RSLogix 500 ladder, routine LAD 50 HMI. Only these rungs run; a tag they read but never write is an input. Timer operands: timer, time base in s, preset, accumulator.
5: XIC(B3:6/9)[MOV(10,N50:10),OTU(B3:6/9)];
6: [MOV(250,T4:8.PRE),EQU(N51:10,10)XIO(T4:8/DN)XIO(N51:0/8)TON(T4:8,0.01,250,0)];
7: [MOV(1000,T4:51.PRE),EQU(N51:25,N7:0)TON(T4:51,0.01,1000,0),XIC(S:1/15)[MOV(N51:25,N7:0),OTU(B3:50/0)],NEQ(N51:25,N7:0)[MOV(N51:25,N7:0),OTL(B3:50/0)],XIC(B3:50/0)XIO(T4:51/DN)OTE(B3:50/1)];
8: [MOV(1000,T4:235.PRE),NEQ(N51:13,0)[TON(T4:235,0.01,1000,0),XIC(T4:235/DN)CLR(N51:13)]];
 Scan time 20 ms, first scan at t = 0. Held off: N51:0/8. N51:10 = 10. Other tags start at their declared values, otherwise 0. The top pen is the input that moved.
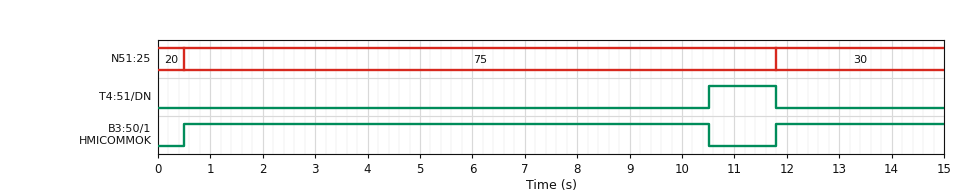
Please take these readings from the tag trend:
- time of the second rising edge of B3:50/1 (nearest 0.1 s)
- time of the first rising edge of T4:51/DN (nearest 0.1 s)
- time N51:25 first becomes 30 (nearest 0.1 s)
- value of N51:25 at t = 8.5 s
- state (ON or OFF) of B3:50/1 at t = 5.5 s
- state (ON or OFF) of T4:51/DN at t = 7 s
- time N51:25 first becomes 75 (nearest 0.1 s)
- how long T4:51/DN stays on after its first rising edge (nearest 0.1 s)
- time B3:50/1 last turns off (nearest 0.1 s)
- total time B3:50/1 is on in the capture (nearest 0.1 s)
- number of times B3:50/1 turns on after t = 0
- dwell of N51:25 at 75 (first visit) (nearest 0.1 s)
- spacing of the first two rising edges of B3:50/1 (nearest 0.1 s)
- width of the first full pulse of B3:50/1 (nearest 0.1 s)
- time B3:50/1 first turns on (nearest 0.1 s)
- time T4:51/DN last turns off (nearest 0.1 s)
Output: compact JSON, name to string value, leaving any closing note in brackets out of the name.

{"time of the second rising edge of B3:50/1": "11.8 s", "time of the first rising edge of T4:51/DN": "10.5 s", "time N51:25 first becomes 30": "11.8 s", "value of N51:25 at t = 8.5 s": "75", "state (ON or OFF) of B3:50/1 at t = 5.5 s": "ON", "state (ON or OFF) of T4:51/DN at t = 7 s": "OFF", "time N51:25 first becomes 75": "0.5 s", "how long T4:51/DN stays on after its first rising edge": "1.3 s", "time B3:50/1 last turns off": "10.5 s", "total time B3:50/1 is on in the capture": "13.2 s", "number of times B3:50/1 turns on after t = 0": "2", "dwell of N51:25 at 75 (first visit)": "11.3 s", "spacing of the first two rising edges of B3:50/1": "11.3 s", "width of the first full pulse of B3:50/1": "10.0 s", "time B3:50/1 first turns on": "0.5 s", "time T4:51/DN last turns off": "11.8 s"}
